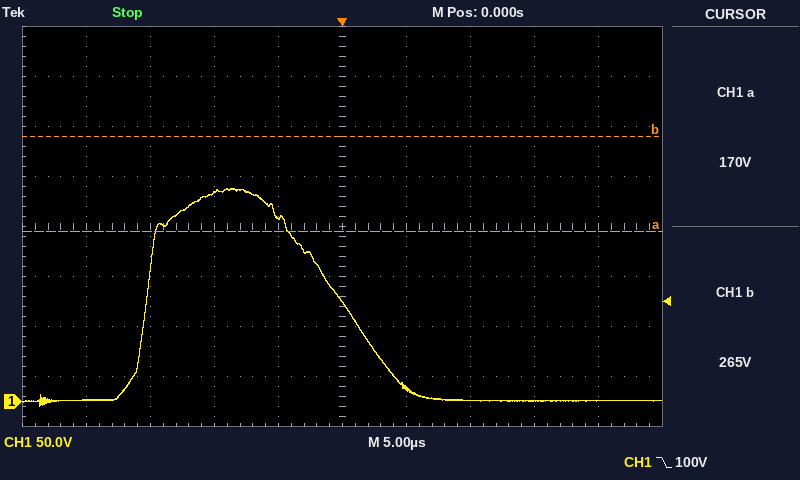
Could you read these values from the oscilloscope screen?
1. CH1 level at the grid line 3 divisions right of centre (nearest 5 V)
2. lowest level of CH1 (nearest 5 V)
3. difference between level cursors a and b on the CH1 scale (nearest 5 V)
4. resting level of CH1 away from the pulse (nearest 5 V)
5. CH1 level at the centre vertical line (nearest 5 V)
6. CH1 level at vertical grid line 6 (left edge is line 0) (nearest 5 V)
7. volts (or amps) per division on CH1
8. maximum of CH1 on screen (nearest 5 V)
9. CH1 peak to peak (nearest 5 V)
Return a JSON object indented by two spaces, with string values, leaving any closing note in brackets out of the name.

{
  "CH1 level at the grid line 3 divisions right of centre": "0 V",
  "lowest level of CH1": "-5 V",
  "difference between level cursors a and b on the CH1 scale": "95 V",
  "resting level of CH1 away from the pulse": "0 V",
  "CH1 level at the centre vertical line": "100 V",
  "CH1 level at vertical grid line 6 (left edge is line 0)": "15 V",
  "volts (or amps) per division on CH1": "50 V",
  "maximum of CH1 on screen": "215 V",
  "CH1 peak to peak": "220 V"
}
